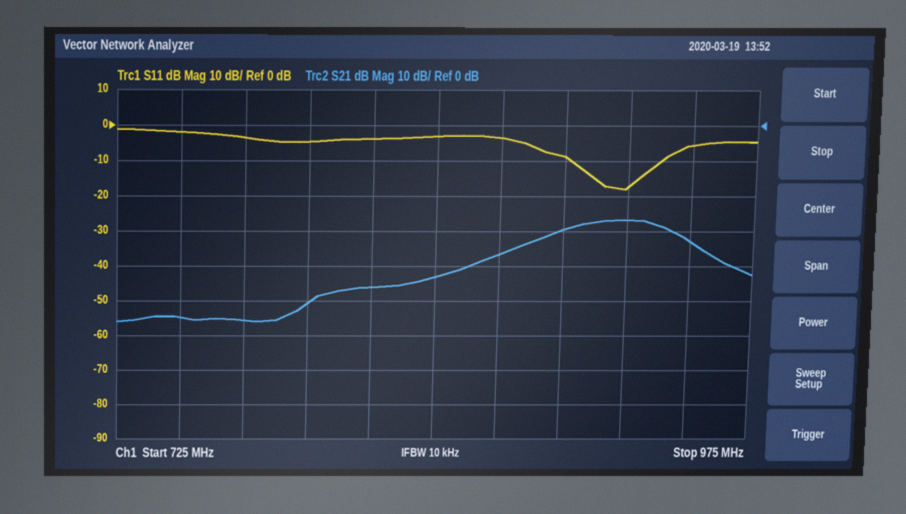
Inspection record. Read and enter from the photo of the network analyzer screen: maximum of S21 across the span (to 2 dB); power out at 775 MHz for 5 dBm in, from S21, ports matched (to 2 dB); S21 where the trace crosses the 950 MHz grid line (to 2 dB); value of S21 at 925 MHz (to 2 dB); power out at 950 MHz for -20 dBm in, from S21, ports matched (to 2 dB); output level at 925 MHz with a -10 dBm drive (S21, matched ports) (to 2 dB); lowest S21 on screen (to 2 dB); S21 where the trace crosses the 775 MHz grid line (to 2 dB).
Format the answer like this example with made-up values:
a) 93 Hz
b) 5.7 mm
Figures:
a) -26 dB
b) -50 dBm
c) -32 dB
d) -26 dB
e) -52 dBm
f) -36 dBm
g) -56 dB
h) -56 dB
